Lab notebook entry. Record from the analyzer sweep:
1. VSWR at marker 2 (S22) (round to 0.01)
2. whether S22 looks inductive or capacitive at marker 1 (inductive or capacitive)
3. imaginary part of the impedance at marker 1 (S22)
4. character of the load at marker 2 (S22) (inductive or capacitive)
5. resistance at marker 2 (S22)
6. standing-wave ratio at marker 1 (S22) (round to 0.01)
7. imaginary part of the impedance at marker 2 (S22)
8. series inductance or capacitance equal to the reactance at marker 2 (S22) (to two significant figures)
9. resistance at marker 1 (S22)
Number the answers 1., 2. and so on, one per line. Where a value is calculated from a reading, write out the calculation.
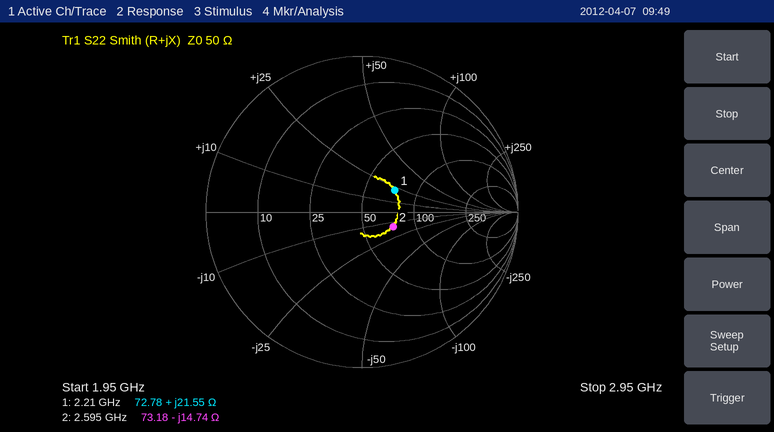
1. 1.57
2. inductive
3. +21.55 Ω
4. capacitive
5. 73.18 Ω
6. 1.67
7. -14.74 Ω
8. C = 1/(2π × 2.595 GHz × 14.74 Ω) ≈ 4.2 pF
9. 72.78 Ω
